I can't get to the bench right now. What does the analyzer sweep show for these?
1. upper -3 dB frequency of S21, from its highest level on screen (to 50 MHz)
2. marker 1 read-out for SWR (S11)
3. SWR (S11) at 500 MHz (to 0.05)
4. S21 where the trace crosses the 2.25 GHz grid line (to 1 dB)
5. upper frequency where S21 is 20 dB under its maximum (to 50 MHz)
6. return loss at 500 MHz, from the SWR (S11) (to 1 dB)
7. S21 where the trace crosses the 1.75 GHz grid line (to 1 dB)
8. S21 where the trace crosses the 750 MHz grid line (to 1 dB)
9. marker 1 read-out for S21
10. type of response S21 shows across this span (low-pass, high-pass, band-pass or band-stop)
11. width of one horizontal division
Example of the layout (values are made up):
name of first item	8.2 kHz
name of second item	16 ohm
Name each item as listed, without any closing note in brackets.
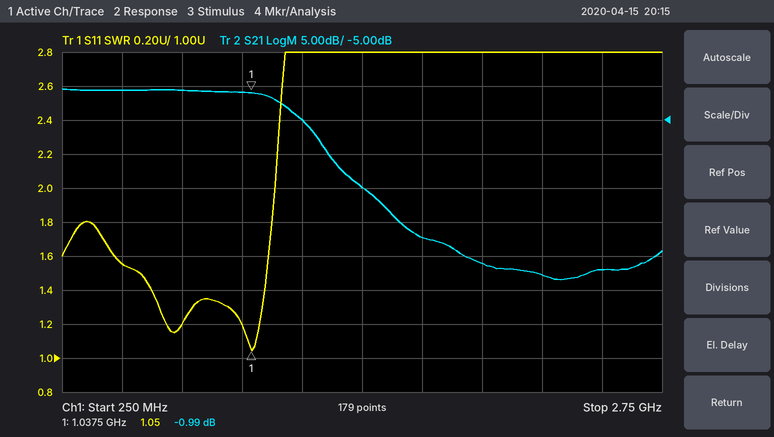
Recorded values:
upper -3 dB frequency of S21, from its highest level on screen	1.20 GHz
marker 1 read-out for SWR	1.05
SWR (S11) at 500 MHz	1.55
S21 where the trace crosses the 2.25 GHz grid line	-28 dB
upper frequency where S21 is 20 dB under its maximum	1.65 GHz
return loss at 500 MHz, from the SWR (S11)	13 dB
S21 where the trace crosses the 1.75 GHz grid line	-22 dB
S21 where the trace crosses the 750 MHz grid line	-1 dB
marker 1 read-out for S21	-0.99 dB
type of response S21 shows across this span	low-pass
width of one horizontal division	250 MHz
